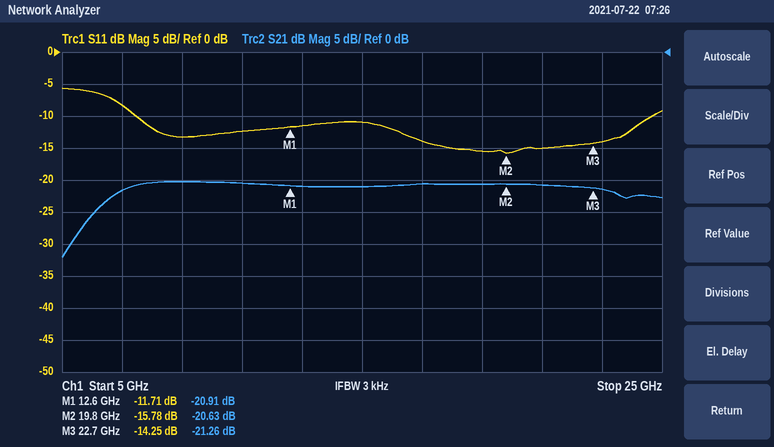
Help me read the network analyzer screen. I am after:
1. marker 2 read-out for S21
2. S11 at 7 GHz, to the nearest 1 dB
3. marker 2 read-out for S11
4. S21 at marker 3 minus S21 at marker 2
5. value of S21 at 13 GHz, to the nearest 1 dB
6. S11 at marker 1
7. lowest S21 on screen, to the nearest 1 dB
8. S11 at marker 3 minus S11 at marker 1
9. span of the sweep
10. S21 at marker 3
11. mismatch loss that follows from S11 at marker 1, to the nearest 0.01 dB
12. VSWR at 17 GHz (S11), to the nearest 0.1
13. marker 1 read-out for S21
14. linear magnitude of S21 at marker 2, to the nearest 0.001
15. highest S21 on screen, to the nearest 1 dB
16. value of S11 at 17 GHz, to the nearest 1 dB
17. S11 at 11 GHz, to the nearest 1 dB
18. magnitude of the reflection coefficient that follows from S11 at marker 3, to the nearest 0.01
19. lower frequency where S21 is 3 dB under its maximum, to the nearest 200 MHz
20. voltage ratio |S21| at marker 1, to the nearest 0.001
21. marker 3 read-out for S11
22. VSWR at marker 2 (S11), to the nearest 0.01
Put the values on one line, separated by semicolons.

-20.63 dB; -8 dB; -15.78 dB; -0.63 dB; -21 dB; -11.71 dB; -32 dB; -2.54 dB; 20 GHz; -21.26 dB; 0.30 dB; 1.5; -20.91 dB; 0.093; -20 dB; -14 dB; -12 dB; 0.19; 6.4 GHz; 0.090; -14.25 dB; 1.39
